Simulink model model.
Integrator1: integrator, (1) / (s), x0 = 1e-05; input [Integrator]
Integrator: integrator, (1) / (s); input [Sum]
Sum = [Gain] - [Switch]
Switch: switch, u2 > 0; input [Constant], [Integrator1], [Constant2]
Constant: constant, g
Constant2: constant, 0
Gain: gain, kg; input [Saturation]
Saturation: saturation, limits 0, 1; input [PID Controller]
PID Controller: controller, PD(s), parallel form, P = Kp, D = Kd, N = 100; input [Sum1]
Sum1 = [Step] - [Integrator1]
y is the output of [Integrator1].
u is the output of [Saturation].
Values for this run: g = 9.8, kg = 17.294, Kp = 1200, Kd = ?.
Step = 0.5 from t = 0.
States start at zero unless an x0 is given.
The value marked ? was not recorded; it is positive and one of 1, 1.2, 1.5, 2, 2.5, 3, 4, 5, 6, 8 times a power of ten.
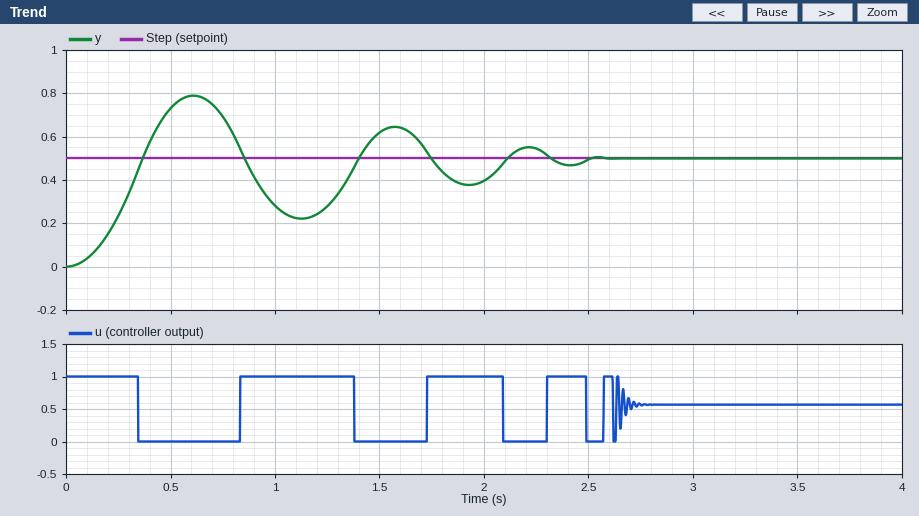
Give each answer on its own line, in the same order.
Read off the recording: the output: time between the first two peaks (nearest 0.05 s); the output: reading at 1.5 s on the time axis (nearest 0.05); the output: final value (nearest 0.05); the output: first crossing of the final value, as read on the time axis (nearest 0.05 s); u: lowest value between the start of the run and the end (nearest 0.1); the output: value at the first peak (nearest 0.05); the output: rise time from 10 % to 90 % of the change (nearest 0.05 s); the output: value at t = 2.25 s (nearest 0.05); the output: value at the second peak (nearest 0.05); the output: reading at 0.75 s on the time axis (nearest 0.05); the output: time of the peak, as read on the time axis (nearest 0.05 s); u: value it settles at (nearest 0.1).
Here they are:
0.95 s
0.60
0.50
0.35 s
0.0
0.80
0.25 s
0.55
0.65
0.70
0.60 s
0.6
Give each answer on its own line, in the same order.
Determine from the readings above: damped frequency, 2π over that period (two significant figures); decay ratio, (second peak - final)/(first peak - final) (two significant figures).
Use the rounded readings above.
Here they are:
6.6 rad/s
0.50
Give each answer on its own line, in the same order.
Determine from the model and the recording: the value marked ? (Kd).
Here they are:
25
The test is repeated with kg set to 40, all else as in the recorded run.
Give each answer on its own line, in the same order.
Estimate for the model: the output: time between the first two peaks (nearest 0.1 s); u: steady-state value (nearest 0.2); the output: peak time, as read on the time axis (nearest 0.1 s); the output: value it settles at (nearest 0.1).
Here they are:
1.1 s
0.2
0.7 s
0.5
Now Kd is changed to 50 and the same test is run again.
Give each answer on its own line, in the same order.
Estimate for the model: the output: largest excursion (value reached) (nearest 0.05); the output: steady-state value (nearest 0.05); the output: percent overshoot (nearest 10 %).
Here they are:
0.70
0.50
40 %
